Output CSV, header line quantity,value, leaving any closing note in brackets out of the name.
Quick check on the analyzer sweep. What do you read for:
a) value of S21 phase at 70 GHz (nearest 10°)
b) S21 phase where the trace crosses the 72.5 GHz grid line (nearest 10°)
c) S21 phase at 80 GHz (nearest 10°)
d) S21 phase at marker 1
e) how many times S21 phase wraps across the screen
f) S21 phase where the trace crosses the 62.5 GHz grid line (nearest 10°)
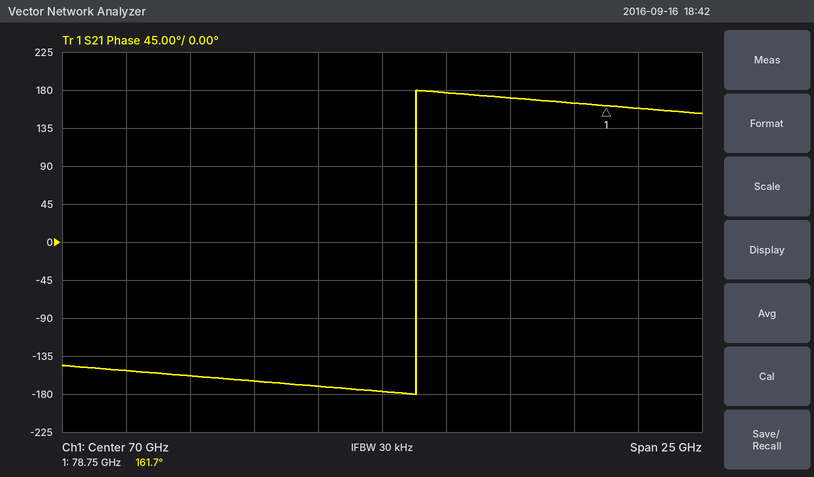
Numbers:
quantity,value
value of S21 phase at 70 GHz,-180°
S21 phase where the trace crosses the 72.5 GHz grid line,180°
S21 phase at 80 GHz,160°
S21 phase at marker 1,161.7°
how many times S21 phase wraps across the screen,1
S21 phase where the trace crosses the 62.5 GHz grid line,-160°
